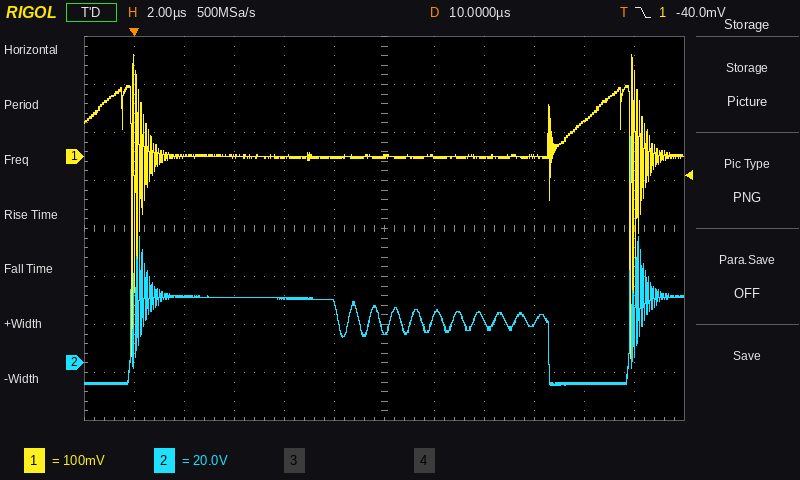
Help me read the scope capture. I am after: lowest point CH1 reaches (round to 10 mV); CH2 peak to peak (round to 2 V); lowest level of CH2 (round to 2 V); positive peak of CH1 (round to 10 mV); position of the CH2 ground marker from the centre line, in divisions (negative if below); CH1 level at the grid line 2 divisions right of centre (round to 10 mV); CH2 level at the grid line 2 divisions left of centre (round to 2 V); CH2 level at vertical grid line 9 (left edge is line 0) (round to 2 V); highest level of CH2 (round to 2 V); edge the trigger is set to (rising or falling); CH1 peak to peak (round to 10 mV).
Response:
-420 mV
104 V
-10 V
210 mV
-2.8 div
0 mV
26 V
16 V
94 V
falling
630 mV
